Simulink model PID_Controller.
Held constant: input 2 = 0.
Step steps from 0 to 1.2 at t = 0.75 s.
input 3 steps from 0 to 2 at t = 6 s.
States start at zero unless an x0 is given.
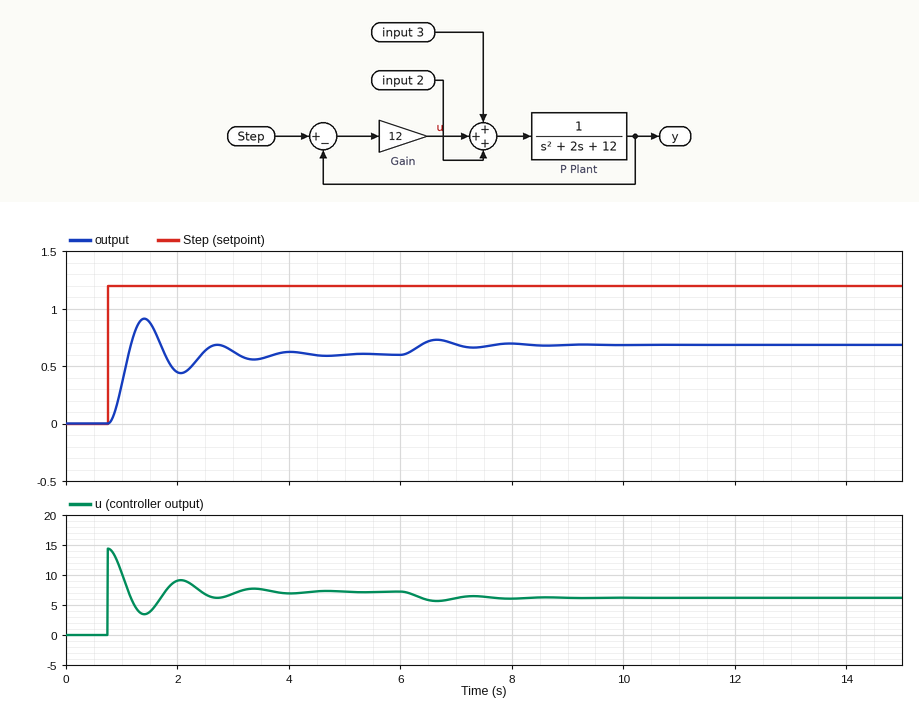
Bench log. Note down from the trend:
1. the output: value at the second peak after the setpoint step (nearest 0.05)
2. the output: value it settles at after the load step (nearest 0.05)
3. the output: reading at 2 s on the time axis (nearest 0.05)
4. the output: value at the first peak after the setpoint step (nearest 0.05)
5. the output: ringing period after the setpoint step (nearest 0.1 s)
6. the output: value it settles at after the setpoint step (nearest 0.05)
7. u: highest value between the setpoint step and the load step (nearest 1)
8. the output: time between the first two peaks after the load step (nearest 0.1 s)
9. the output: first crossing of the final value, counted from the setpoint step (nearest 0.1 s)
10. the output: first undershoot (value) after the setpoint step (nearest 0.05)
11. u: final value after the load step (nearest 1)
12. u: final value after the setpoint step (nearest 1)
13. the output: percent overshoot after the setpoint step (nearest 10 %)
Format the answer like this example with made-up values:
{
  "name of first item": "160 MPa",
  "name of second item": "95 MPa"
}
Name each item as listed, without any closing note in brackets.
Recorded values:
{
  "the output: value at the second peak after the setpoint step": "0.70",
  "the output: value it settles at after the load step": "0.70",
  "the output: reading at 2 s on the time axis": "0.45",
  "the output: value at the first peak after the setpoint step": "0.90",
  "the output: ringing period after the setpoint step": "1.3 s",
  "the output: value it settles at after the setpoint step": "0.60",
  "u: highest value between the setpoint step and the load step": "14",
  "the output: time between the first two peaks after the load step": "1.3 s",
  "the output: first crossing of the final value, counted from the setpoint step": "0.4 s",
  "the output: first undershoot (value) after the setpoint step": "0.45",
  "u: final value after the load step": "6",
  "u: final value after the setpoint step": "7",
  "the output: percent overshoot after the setpoint step": "50 %"
}
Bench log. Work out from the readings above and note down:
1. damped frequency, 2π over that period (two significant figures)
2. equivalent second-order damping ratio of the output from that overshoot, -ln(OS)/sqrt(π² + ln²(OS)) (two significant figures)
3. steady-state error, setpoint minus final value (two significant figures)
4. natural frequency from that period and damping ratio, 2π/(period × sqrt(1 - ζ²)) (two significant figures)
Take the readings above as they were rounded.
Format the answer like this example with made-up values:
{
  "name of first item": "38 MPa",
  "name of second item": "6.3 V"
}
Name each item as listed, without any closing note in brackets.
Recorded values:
{
  "damped frequency, 2π over that period": "4.8 rad/s",
  "equivalent second-order damping ratio of the output from that overshoot, -ln(OS)/sqrt(π² + ln²(OS))": "0.22",
  "steady-state error, setpoint minus final value": "0.60",
  "natural frequency from that period and damping ratio, 2π/(period × sqrt(1 - ζ²))": "5.0 rad/s"
}
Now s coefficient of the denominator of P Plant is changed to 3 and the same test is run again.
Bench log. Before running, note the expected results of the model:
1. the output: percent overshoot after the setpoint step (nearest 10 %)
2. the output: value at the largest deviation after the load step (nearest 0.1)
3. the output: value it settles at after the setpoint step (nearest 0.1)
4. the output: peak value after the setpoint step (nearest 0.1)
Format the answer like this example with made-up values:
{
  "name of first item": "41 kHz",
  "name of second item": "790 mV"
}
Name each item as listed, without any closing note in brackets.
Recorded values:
{
  "the output: percent overshoot after the setpoint step": "40 %",
  "the output: value at the largest deviation after the load step": "0.7",
  "the output: value it settles at after the setpoint step": "0.6",
  "the output: peak value after the setpoint step": "0.8"
}
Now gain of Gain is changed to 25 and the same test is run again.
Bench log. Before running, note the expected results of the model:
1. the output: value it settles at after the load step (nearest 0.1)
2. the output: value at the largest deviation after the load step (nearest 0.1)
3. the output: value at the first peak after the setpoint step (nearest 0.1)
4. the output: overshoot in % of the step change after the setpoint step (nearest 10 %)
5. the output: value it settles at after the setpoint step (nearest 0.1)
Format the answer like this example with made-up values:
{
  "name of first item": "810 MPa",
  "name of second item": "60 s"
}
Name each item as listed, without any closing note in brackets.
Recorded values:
{
  "the output: value it settles at after the load step": "0.9",
  "the output: value at the largest deviation after the load step": "0.9",
  "the output: value at the first peak after the setpoint step": "1.3",
  "the output: overshoot in % of the step change after the setpoint step": "60 %",
  "the output: value it settles at after the setpoint step": "0.8"
}
